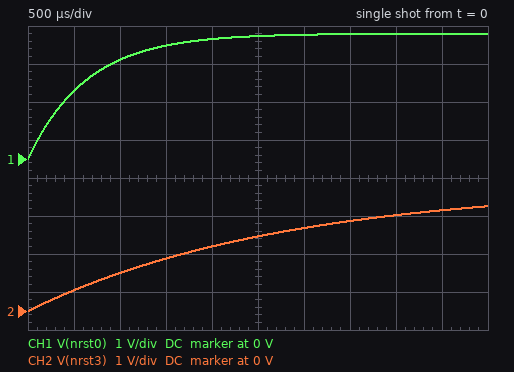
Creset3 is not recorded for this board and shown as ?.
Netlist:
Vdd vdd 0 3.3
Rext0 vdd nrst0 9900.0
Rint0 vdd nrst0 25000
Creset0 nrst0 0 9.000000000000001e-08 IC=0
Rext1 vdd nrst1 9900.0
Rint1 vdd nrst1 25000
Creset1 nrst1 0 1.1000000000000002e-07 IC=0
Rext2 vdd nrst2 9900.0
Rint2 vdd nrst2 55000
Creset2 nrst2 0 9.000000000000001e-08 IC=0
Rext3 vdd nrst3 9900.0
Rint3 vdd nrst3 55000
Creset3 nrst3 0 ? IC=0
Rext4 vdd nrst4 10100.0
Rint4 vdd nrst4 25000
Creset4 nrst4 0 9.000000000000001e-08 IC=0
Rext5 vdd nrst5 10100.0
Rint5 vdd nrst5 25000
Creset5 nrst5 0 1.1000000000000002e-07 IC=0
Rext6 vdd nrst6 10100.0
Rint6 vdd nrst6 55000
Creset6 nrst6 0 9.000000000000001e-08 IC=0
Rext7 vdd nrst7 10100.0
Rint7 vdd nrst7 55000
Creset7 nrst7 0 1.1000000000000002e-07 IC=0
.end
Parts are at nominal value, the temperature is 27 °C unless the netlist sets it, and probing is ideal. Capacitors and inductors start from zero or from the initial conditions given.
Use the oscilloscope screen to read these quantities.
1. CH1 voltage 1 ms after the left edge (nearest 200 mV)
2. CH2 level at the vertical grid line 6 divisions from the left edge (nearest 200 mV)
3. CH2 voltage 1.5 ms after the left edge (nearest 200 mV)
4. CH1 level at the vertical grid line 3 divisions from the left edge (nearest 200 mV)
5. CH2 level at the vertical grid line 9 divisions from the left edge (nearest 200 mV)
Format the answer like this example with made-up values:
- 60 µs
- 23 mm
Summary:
- 2.6 V
- 2.2 V
- 1.4 V
- 3.0 V
- 2.6 V
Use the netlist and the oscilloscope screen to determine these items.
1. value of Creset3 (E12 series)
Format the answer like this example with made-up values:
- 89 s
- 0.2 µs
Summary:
- 330 nF
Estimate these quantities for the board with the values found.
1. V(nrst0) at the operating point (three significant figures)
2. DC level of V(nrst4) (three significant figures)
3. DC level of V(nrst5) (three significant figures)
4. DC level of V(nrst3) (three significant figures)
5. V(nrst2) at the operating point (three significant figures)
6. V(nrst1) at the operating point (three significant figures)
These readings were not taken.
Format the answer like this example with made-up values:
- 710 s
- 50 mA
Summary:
- 3.30 V
- 3.30 V
- 3.30 V
- 3.30 V
- 3.30 V
- 3.30 V
